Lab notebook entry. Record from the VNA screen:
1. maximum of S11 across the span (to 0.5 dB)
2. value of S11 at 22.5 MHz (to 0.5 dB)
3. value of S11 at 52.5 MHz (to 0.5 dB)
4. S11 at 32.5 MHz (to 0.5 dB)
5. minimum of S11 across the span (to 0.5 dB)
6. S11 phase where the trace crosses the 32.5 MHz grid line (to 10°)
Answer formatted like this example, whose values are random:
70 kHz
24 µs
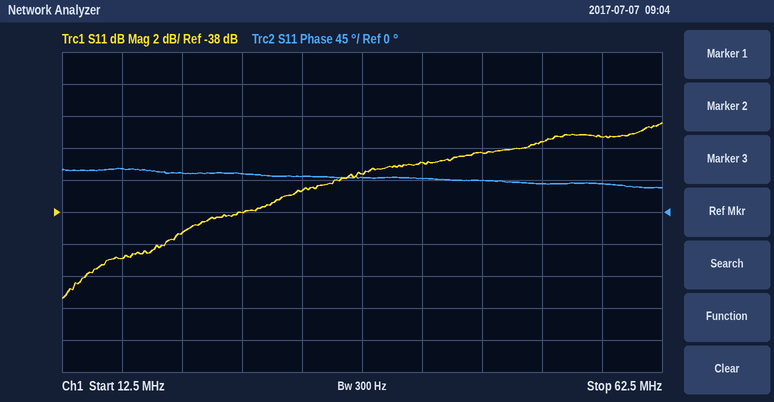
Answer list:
-32.5 dB
-39.5 dB
-33.5 dB
-36.5 dB
-43.5 dB
50°
